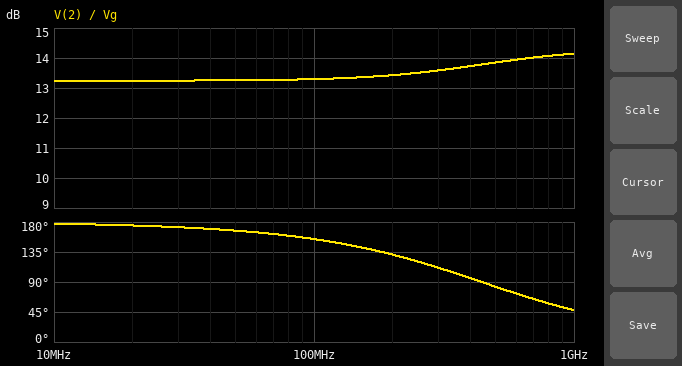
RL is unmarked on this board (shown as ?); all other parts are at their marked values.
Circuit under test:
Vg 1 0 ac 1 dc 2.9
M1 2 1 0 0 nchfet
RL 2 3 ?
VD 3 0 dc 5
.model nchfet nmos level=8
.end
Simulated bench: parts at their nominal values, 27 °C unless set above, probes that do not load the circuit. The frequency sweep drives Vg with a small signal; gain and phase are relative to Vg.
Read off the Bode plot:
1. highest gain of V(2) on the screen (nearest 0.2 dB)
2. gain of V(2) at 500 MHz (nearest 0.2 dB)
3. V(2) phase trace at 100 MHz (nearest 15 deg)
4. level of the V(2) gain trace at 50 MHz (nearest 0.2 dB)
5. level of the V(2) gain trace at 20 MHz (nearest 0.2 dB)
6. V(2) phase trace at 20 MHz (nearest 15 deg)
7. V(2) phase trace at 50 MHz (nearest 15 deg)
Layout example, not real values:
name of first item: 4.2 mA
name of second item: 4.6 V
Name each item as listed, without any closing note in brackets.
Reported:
highest gain of V(2) on the screen: 14.2 dB
gain of V(2) at 500 MHz: 13.8 dB
V(2) phase trace at 100 MHz: 150 deg
level of the V(2) gain trace at 50 MHz: 13.2 dB
level of the V(2) gain trace at 20 MHz: 13.2 dB
V(2) phase trace at 20 MHz: 180 deg
V(2) phase trace at 50 MHz: 165 deg
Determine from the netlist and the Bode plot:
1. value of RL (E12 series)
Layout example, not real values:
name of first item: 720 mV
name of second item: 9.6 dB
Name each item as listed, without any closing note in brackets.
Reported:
value of RL: 150 kΩ
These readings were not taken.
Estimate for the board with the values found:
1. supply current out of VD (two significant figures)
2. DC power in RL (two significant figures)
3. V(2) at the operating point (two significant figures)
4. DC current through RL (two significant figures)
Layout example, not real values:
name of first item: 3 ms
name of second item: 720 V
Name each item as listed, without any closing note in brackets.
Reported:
supply current out of VD: 29 µA
DC power in RL: 130 µW
V(2) at the operating point: 650 mV
DC current through RL: 29 µA
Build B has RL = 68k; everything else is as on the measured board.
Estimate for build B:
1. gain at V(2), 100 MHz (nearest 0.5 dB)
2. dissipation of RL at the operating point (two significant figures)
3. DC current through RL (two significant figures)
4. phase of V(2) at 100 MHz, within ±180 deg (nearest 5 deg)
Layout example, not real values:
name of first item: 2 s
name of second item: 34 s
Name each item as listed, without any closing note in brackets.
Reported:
gain at V(2), 100 MHz: 10.0 dB
dissipation of RL at the operating point: 62 µW
DC current through RL: 30 µA
phase of V(2) at 100 MHz, within ±180 deg: 165 deg
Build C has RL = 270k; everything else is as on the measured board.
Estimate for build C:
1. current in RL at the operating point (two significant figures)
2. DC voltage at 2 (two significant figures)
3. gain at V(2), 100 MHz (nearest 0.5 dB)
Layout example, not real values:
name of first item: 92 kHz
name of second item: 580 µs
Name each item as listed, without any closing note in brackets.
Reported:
current in RL at the operating point: 18 µA
DC voltage at 2: 220 mV
gain at V(2), 100 MHz: -8.5 dB
